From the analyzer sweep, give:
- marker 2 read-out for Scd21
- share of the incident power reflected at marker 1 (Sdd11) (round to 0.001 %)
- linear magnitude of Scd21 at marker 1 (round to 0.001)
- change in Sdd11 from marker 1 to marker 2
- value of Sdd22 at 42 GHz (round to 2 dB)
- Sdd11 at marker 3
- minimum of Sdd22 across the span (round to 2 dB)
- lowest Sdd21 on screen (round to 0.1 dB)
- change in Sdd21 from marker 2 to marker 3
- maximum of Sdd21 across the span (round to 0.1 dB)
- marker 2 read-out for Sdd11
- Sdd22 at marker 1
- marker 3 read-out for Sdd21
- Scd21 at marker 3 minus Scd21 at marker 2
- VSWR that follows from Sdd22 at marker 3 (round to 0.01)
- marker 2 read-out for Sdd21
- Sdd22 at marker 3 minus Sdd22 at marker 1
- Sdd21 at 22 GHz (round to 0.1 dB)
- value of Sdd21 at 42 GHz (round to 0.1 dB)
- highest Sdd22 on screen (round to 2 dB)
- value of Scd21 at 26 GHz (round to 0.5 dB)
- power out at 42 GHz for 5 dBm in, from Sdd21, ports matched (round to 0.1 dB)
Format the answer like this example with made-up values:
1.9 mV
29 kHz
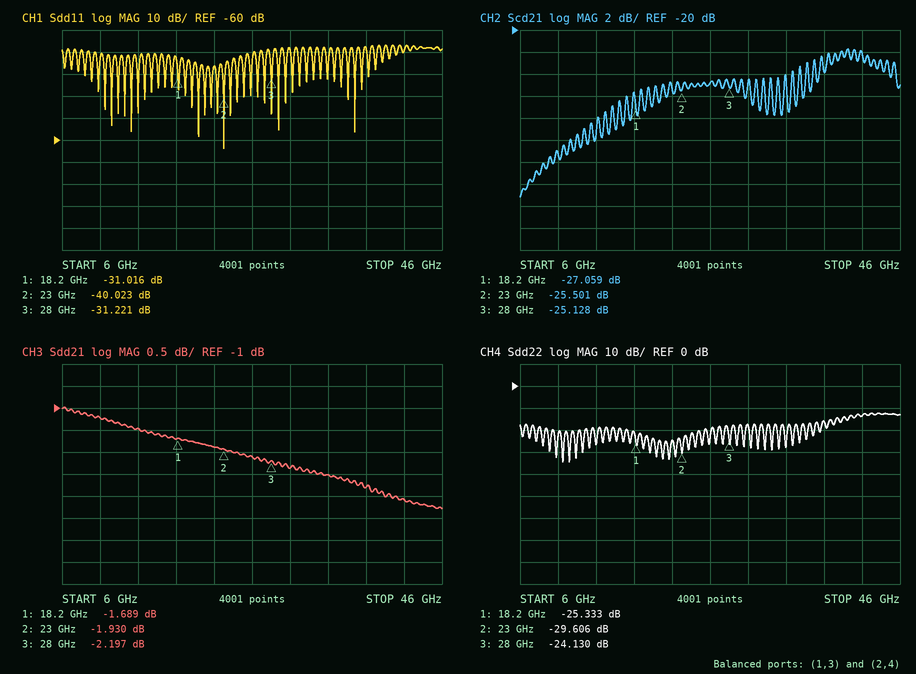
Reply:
-25.501 dB
0.079 %
0.044
-9.007 dB
-14 dB
-31.221 dB
-34 dB
-3.3 dB
-0.267 dB
-1.0 dB
-40.023 dB
-25.333 dB
-2.197 dB
0.373 dB
1.13
-1.930 dB
1.203 dB
-1.9 dB
-3.1 dB
-12 dB
-25.0 dB
1.9 dBm
